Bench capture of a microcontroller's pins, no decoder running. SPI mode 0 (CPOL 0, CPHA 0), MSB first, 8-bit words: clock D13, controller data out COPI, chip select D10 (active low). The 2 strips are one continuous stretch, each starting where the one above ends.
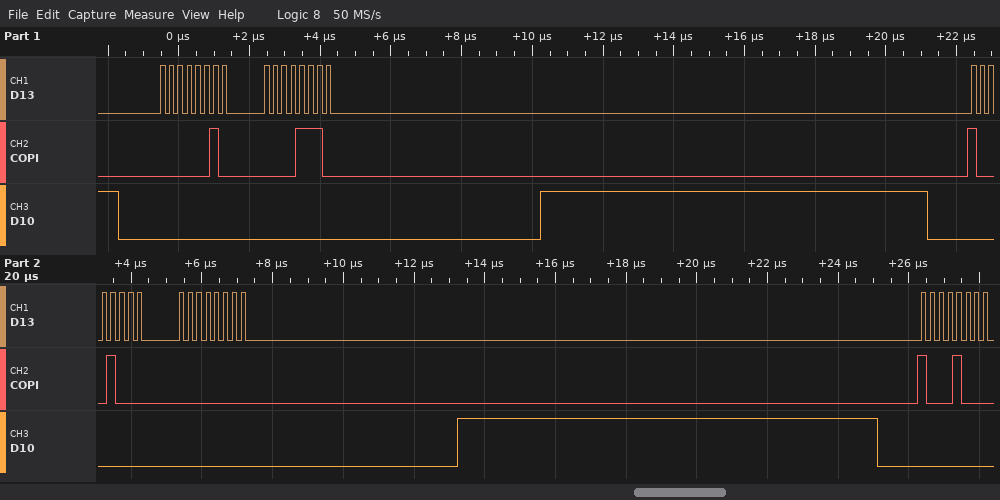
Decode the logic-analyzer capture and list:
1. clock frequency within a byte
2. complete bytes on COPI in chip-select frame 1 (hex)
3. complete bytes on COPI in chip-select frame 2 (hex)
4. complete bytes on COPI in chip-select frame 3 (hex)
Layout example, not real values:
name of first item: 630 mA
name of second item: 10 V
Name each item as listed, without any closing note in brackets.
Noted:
clock frequency within a byte: 4 MHz
complete bytes on COPI in chip-select frame 1: 02 0E
complete bytes on COPI in chip-select frame 2: 88 00
complete bytes on COPI in chip-select frame 3: 88
